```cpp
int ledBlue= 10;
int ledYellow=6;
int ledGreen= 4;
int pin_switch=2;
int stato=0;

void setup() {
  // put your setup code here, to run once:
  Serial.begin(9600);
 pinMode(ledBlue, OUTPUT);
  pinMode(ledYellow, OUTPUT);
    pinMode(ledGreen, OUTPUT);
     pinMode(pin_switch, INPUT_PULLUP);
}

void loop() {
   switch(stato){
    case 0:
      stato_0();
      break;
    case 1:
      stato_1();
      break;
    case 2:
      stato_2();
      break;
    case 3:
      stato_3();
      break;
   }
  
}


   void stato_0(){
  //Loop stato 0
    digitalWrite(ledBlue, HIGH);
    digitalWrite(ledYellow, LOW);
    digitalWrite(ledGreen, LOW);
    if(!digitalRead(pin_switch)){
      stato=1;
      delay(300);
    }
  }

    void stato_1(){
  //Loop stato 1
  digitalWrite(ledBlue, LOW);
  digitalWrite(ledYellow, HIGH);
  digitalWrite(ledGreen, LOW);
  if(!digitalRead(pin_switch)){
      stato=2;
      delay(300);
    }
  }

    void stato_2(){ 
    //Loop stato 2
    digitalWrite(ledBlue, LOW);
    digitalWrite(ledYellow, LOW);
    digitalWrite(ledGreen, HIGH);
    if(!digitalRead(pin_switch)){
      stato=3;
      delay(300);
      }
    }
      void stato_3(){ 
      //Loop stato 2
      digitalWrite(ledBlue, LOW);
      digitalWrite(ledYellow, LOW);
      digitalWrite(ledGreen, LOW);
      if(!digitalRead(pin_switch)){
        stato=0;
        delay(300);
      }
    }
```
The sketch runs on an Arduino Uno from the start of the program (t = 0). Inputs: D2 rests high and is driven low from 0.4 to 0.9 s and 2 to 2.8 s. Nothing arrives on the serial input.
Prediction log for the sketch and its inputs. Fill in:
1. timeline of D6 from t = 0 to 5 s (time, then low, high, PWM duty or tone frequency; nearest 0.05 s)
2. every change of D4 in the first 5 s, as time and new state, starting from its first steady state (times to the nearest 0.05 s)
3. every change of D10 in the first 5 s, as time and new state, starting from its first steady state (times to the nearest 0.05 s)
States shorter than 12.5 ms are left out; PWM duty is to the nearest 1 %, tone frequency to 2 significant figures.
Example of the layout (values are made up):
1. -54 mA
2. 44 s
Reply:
1. 0 s low; 0.7 s high; 1 s low; 2.9 s high
2. 0 s low; 1 s high; 2.3 s low
3. 0 s high; 0.7 s low; 2.6 s high; 2.9 s low
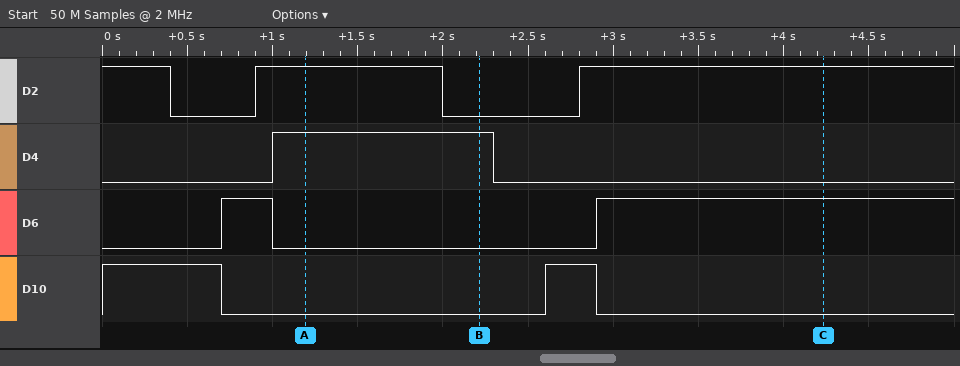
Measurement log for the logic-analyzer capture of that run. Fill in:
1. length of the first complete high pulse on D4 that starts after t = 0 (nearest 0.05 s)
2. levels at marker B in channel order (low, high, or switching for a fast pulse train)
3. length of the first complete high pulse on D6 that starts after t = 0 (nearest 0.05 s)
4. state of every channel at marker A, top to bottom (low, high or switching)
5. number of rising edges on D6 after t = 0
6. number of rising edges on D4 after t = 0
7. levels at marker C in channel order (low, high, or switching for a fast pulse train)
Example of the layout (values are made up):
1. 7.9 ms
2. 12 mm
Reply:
1. 1.30 s
2. D2 low, D4 high, D6 low, D10 low
3. 0.30 s
4. D2 high, D4 high, D6 low, D10 low
5. 2
6. 1
7. D2 high, D4 low, D6 high, D10 low
